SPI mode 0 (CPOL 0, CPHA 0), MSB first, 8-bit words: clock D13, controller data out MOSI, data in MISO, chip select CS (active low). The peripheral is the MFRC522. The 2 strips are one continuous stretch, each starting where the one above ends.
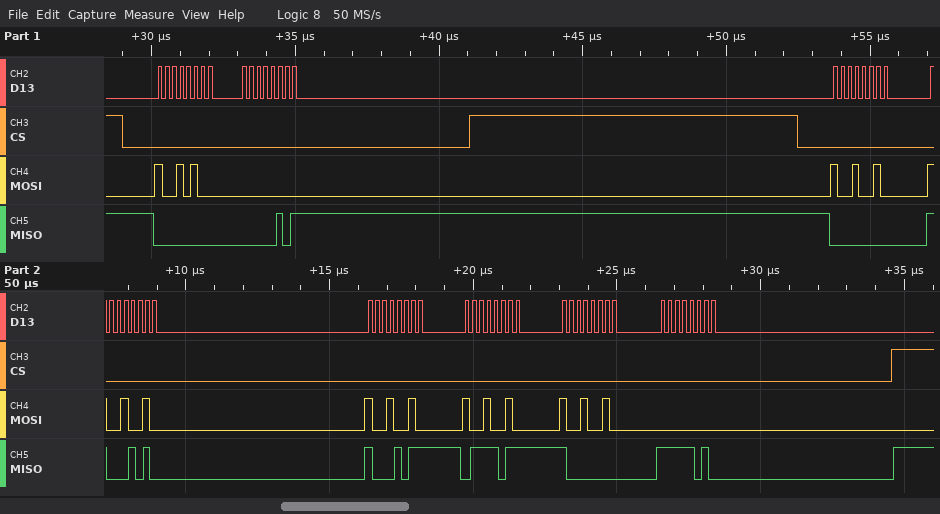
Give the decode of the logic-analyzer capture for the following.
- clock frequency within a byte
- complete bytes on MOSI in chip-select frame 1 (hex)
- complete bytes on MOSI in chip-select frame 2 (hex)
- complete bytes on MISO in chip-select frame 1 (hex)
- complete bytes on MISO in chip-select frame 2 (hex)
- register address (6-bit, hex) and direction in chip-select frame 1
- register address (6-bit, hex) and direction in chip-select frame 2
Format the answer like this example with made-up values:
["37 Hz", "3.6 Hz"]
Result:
["4 MHz", "94 00", "92 92 92 92 92 00", "00 05", "00 8A 8B 7B 80 FA", "0x0A read", "0x09 read"]
